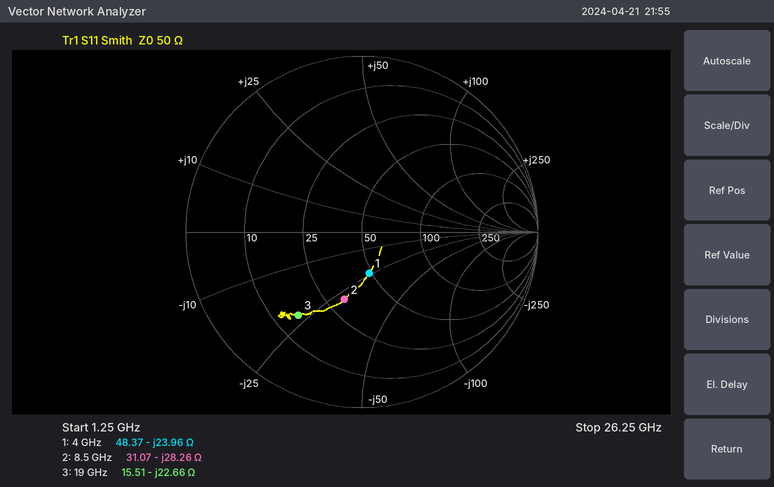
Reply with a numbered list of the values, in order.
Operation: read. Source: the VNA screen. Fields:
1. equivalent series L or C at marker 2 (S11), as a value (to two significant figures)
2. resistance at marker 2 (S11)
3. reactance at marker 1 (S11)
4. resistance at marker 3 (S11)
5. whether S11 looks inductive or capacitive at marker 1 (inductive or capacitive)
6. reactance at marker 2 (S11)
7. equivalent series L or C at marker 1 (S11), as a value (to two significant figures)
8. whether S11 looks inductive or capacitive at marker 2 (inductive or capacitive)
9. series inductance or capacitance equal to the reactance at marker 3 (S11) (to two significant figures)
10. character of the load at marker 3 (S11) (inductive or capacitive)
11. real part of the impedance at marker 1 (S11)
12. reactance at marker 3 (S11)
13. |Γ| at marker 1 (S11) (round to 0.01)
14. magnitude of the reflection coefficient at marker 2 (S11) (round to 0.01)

1. 660 fF
2. 31.07 Ω
3. -23.96 Ω
4. 15.51 Ω
5. capacitive
6. -28.26 Ω
7. 1.7 pF
8. capacitive
9. 370 fF
10. capacitive
11. 48.37 Ω
12. -22.66 Ω
13. 0.24
14. 0.40
